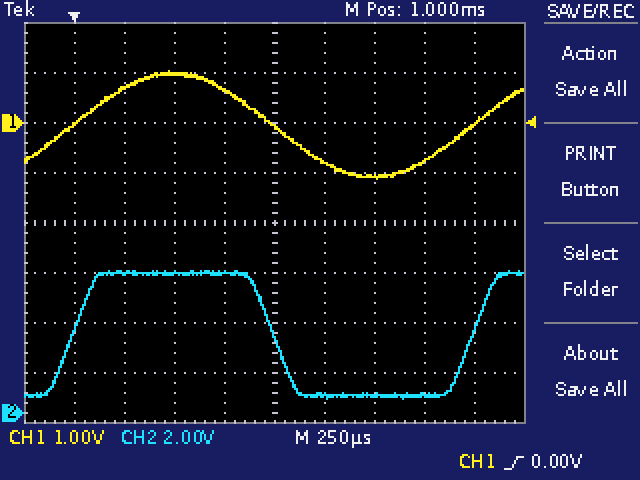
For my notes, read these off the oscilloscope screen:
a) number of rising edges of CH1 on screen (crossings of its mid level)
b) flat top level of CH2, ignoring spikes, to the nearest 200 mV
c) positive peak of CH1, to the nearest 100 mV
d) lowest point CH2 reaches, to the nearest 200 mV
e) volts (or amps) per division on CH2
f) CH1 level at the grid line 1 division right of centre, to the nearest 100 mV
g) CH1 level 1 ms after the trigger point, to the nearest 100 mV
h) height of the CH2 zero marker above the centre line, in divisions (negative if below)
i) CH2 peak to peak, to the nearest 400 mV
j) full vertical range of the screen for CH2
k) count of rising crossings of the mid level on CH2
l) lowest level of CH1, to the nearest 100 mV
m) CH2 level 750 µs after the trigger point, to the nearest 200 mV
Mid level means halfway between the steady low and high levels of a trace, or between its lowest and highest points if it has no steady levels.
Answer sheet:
2
5.6 V
1.0 V
600 mV
2 V
-800 mV
-100 mV
-3.8 div
5.2 V
16 V
2
-1.1 V
5.6 V
